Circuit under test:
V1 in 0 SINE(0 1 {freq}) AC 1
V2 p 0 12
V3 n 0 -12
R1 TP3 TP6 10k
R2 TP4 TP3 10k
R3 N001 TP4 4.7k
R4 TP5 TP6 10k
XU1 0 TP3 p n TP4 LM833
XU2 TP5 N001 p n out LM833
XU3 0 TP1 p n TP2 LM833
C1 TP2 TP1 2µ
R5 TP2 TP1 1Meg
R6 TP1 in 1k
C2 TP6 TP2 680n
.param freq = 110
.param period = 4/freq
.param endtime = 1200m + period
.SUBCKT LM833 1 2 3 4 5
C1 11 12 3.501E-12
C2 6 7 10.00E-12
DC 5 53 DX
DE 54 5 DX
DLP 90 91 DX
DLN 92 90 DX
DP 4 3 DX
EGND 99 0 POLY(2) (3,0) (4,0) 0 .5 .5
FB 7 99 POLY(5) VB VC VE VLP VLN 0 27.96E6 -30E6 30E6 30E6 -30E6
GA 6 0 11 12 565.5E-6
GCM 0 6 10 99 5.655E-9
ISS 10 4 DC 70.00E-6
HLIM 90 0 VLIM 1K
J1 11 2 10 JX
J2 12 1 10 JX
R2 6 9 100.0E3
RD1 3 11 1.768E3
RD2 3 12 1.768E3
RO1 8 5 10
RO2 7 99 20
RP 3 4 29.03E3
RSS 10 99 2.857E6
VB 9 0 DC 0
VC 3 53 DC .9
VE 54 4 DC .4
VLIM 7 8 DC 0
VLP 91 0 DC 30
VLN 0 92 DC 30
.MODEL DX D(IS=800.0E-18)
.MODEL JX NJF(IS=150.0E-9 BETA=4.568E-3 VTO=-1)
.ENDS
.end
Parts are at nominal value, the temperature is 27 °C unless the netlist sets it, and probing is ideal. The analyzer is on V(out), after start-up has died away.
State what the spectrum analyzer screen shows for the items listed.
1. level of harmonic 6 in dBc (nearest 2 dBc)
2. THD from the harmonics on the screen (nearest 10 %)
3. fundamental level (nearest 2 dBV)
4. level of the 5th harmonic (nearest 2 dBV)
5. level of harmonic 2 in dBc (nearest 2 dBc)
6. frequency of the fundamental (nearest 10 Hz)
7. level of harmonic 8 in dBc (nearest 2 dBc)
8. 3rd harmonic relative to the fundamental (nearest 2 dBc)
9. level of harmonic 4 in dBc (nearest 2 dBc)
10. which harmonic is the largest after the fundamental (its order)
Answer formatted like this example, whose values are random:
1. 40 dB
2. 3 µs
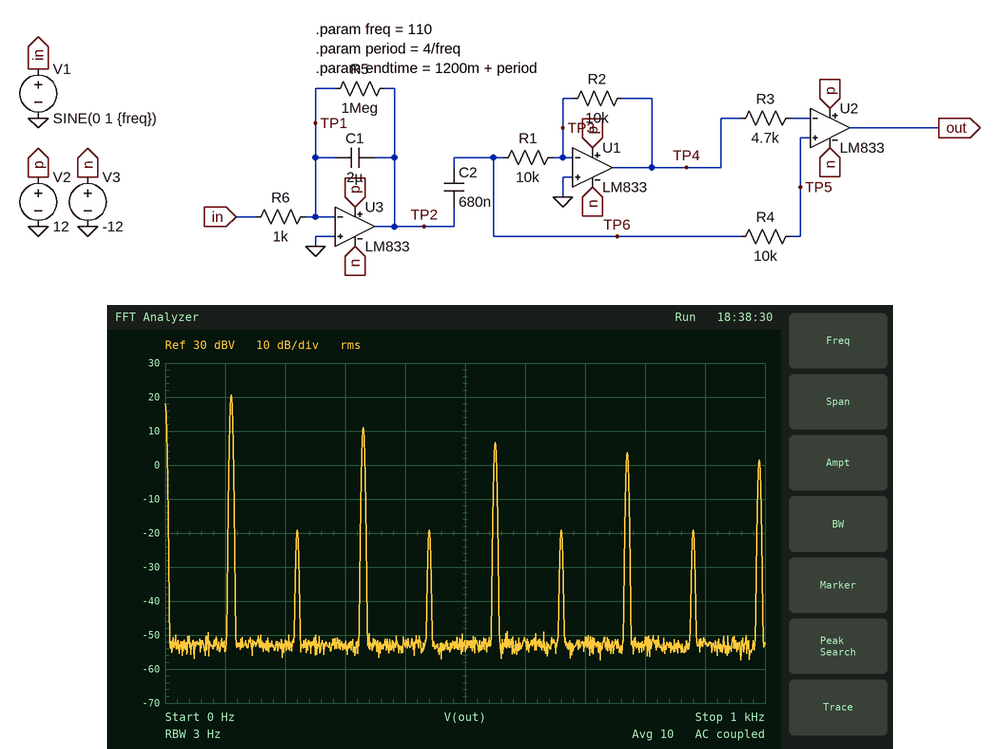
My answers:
1. -40 dBc
2. 40 %
3. 20 dBV
4. 6 dBV
5. -40 dBc
6. 110 Hz
7. -40 dBc
8. -10 dBc
9. -40 dBc
10. 3
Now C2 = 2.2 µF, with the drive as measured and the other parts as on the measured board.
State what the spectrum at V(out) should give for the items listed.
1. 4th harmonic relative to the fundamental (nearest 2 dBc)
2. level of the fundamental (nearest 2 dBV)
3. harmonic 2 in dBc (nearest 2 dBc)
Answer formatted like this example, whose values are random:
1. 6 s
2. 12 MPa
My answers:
1. -36 dBc
2. 20 dBV
3. -36 dBc
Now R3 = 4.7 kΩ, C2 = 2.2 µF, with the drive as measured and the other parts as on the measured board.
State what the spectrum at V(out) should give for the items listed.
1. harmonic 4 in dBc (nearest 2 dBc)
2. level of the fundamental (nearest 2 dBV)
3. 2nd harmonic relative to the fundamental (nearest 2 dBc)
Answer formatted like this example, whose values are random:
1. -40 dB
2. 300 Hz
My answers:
1. -36 dBc
2. 20 dBV
3. -36 dBc
